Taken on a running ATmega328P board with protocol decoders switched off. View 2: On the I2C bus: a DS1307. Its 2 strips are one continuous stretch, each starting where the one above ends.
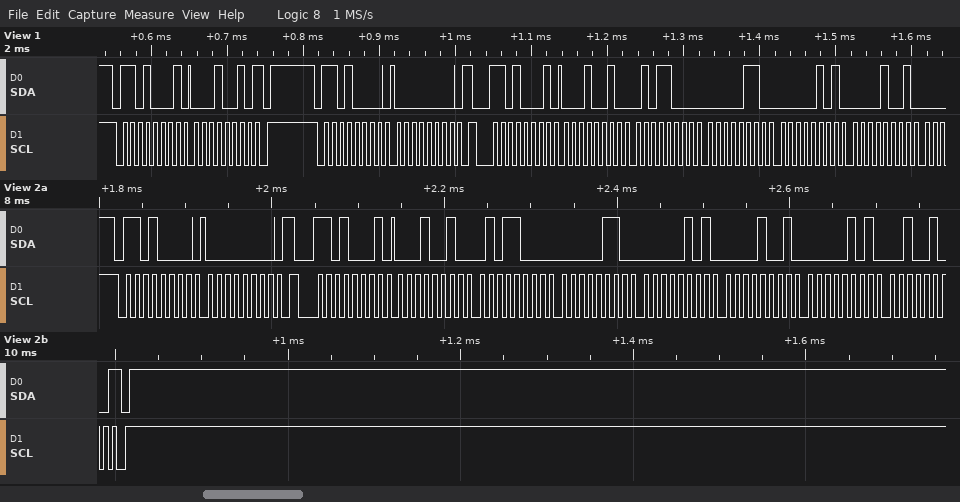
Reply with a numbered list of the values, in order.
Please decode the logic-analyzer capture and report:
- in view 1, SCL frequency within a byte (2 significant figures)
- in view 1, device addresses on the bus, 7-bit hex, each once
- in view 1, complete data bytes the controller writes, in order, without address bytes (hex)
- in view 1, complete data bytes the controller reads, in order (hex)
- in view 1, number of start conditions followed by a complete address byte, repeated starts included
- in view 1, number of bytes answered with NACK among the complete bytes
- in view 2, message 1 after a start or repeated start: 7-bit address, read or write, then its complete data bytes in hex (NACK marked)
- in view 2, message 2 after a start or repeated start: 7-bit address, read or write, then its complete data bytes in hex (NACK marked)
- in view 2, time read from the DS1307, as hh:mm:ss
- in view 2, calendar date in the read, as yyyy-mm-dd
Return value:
1. 100 kHz
2. 0x68
3. 00
4. 12 12 58 06 05 09
5. 3
6. 1
7. 0x68 write: 00
8. 0x68 read: 12 58 06 05 09 05 24 NACK
9. 06:58:12
10. 2024-05-09
